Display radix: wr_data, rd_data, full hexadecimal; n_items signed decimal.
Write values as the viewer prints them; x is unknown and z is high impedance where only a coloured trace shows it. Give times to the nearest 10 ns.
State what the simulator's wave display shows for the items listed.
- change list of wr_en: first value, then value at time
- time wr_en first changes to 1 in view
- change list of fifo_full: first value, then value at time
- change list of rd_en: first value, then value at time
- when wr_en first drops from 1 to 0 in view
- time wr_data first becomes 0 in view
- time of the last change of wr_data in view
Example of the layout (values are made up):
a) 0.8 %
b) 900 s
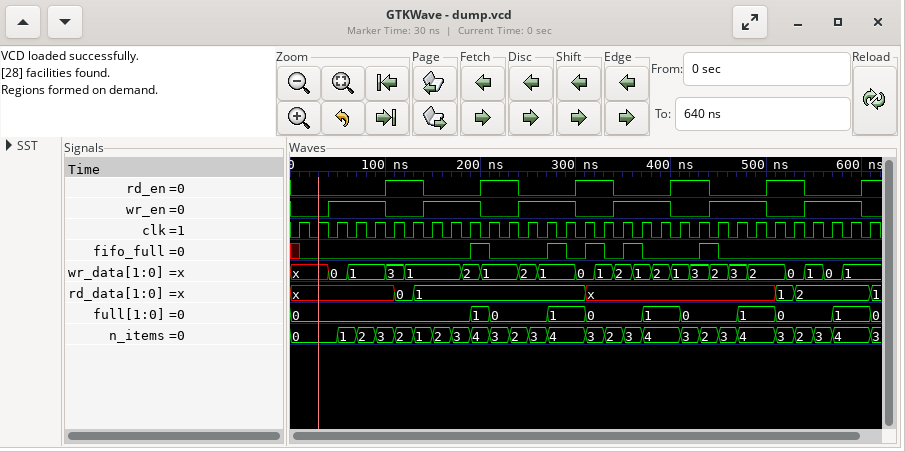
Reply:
a) 0, 1 at 40 ns, 0 at 100 ns, 1 at 140 ns, 0 at 200 ns, 1 at 240 ns, 0 at 300 ns, 1 at 340 ns, 0 at 400 ns, 1 at 440 ns, 0 at 500 ns, 1 at 540 ns, 0 at 600 ns
b) 40 ns
c) x, 0 at 10 ns, 1 at 190 ns, 0 at 210 ns, 1 at 270 ns, 0 at 290 ns, 1 at 310 ns, 0 at 330 ns, 1 at 350 ns, 0 at 370 ns, 1 at 430 ns, 0 at 450 ns
d) 0, 1 at 100 ns, 0 at 140 ns, 1 at 200 ns, 0 at 240 ns, 1 at 300 ns, 0 at 340 ns, 1 at 400 ns, 0 at 440 ns, 1 at 500 ns, 0 at 540 ns, 1 at 600 ns
e) 100 ns
f) 40 ns
g) 580 ns
